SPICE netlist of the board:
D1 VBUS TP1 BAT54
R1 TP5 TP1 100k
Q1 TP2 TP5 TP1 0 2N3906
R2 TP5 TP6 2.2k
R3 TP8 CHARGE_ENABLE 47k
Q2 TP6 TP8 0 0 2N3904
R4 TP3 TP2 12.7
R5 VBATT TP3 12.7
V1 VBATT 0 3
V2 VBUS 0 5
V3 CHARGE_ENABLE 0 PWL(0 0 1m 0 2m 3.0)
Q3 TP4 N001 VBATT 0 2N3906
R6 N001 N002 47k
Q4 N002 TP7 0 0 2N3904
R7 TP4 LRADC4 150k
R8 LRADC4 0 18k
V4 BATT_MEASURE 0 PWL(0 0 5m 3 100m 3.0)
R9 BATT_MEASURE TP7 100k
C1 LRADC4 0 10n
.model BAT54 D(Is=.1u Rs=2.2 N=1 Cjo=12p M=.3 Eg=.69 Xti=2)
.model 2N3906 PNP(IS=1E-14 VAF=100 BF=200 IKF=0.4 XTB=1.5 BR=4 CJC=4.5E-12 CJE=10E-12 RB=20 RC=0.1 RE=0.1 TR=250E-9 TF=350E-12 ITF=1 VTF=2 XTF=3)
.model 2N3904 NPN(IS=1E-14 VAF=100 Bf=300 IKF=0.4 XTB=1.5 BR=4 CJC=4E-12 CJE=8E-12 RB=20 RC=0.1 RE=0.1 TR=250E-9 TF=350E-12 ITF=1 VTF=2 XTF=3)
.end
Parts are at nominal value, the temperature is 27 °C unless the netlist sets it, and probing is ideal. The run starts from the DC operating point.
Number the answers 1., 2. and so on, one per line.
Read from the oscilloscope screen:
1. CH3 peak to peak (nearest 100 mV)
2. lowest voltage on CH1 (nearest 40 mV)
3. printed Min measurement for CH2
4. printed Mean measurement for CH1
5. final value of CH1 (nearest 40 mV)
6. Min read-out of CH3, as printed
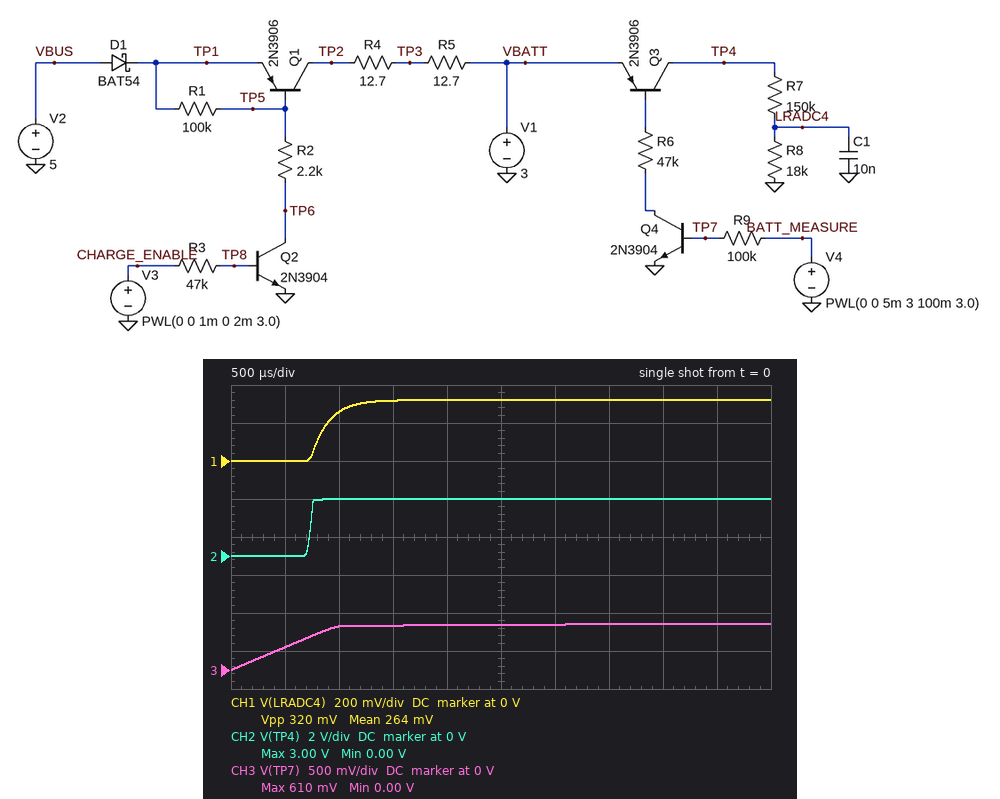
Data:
1. 600 mV
2. 0 V
3. 0.00 V
4. 264 mV
5. 320 mV
6. 0.00 V
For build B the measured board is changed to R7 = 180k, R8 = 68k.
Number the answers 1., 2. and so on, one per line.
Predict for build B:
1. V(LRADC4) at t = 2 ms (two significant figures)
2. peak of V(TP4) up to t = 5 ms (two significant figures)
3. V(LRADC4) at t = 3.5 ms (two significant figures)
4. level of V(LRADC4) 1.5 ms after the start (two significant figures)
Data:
1. 760 mV
2. 3.0 V
3. 820 mV
4. 650 mV
